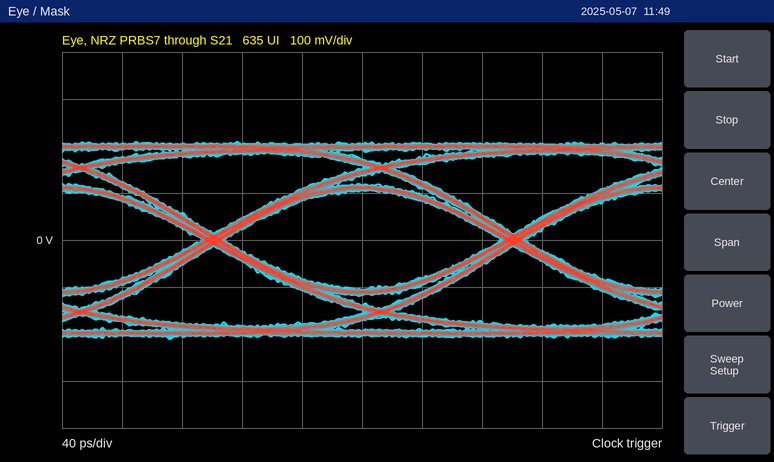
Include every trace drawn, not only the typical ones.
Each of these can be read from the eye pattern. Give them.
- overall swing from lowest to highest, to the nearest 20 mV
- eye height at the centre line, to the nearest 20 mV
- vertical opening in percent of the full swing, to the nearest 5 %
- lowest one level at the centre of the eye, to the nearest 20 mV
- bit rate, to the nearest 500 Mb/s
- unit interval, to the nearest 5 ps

420 mV
220 mV
50 %
100 mV
5.0 Gb/s
200 ps
